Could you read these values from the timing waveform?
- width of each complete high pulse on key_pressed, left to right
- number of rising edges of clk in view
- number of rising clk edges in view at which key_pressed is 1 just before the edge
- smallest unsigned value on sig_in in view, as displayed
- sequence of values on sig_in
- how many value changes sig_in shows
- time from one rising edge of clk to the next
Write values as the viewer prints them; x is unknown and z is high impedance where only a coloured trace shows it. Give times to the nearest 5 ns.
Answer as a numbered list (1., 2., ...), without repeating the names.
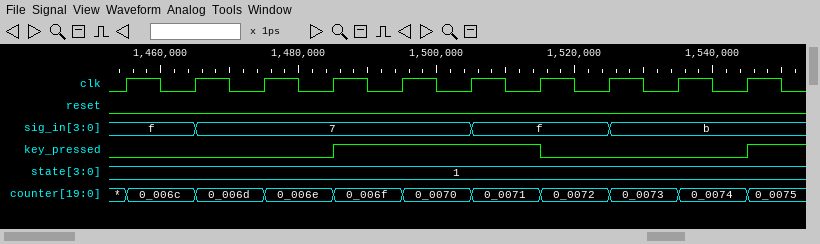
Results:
1. 30 ns
2. 10
3. 3
4. 7
5. f, 7, f, b
6. 3
7. 10 ns
